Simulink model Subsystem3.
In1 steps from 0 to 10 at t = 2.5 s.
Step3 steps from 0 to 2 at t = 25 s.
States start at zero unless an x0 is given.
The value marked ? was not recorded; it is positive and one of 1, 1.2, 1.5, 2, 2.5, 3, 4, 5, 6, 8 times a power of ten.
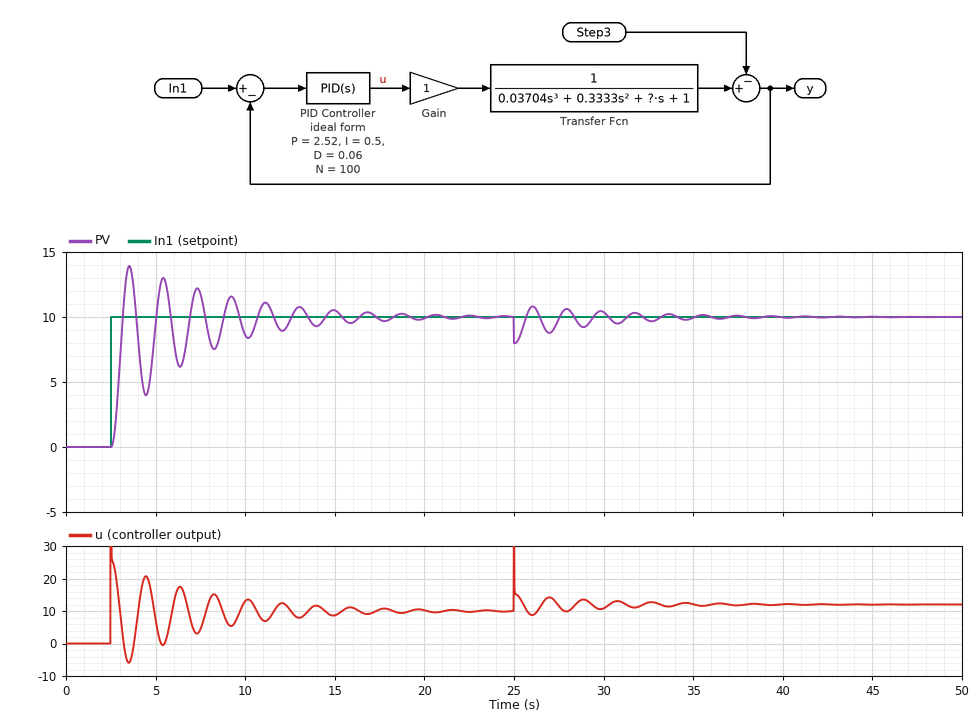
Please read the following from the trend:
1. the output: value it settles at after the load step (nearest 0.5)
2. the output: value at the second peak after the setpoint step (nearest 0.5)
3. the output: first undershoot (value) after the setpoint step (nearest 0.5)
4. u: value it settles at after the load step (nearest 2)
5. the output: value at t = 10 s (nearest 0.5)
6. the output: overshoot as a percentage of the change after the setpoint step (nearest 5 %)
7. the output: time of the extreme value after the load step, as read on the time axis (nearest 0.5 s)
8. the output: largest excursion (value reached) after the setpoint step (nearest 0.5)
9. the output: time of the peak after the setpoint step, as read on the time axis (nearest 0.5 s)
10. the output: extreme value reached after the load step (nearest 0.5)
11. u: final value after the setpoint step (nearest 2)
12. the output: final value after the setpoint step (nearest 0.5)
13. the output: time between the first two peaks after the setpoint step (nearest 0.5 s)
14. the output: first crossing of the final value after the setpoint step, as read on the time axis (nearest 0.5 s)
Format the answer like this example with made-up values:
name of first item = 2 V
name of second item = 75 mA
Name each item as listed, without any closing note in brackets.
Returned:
the output: value it settles at after the load step = 10.0
the output: value at the second peak after the setpoint step = 13.0
the output: first undershoot (value) after the setpoint step = 4.0
u: value it settles at after the load step = 12
the output: value at t = 10 s = 8.5
the output: overshoot as a percentage of the change after the setpoint step = 40 %
the output: time of the extreme value after the load step, as read on the time axis = 25.0 s
the output: largest excursion (value reached) after the setpoint step = 14.0
the output: time of the peak after the setpoint step, as read on the time axis = 3.5 s
the output: extreme value reached after the load step = 8.0
u: final value after the setpoint step = 10
the output: final value after the setpoint step = 10.0
the output: time between the first two peaks after the setpoint step = 2.0 s
the output: first crossing of the final value after the setpoint step, as read on the time axis = 3.0 s
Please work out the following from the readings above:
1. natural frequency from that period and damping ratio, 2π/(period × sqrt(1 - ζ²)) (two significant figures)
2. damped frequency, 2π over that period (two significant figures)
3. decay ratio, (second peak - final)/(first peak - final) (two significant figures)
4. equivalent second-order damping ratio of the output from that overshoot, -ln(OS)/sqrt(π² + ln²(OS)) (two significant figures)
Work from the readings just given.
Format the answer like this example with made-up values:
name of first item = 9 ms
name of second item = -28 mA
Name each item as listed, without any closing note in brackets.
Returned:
natural frequency from that period and damping ratio, 2π/(period × sqrt(1 - ζ²)) = 3.3 rad/s
damped frequency, 2π over that period = 3.1 rad/s
decay ratio, (second peak - final)/(first peak - final) = 0.75
equivalent second-order damping ratio of the output from that overshoot, -ln(OS)/sqrt(π² + ln²(OS)) = 0.28
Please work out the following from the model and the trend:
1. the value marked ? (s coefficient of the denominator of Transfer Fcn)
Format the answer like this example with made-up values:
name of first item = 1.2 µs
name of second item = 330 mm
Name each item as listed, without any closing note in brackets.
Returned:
the value marked ? = 0.5
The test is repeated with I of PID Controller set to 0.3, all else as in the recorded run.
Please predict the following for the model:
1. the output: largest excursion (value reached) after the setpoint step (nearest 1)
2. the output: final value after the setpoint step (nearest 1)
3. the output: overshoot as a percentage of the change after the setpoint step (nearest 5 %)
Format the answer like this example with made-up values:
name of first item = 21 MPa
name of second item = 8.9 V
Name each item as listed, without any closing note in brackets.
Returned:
the output: largest excursion (value reached) after the setpoint step = 13
the output: final value after the setpoint step = 10
the output: overshoot as a percentage of the change after the setpoint step = 30 %
